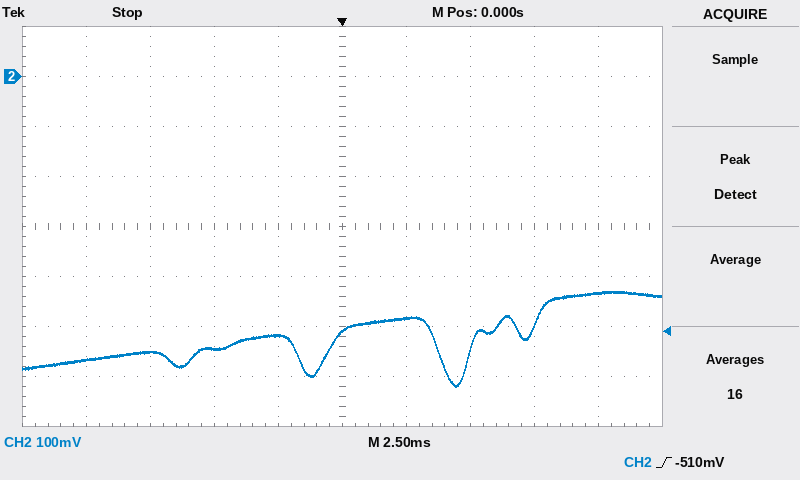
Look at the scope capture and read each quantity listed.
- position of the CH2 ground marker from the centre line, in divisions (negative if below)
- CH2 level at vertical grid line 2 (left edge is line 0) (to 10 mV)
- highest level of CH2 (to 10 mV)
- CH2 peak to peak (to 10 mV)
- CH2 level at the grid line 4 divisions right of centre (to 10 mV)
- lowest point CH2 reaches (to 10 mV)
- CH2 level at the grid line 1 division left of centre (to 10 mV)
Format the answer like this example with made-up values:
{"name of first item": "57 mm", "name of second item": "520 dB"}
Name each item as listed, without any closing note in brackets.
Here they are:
{"position of the CH2 ground marker from the centre line, in divisions": "+3.0 div", "CH2 level at vertical grid line 2 (left edge is line 0)": "-550 mV", "highest level of CH2": "-430 mV", "CH2 peak to peak": "190 mV", "CH2 level at the grid line 4 divisions right of centre": "-430 mV", "lowest point CH2 reaches": "-620 mV", "CH2 level at the grid line 1 division left of centre": "-520 mV"}
